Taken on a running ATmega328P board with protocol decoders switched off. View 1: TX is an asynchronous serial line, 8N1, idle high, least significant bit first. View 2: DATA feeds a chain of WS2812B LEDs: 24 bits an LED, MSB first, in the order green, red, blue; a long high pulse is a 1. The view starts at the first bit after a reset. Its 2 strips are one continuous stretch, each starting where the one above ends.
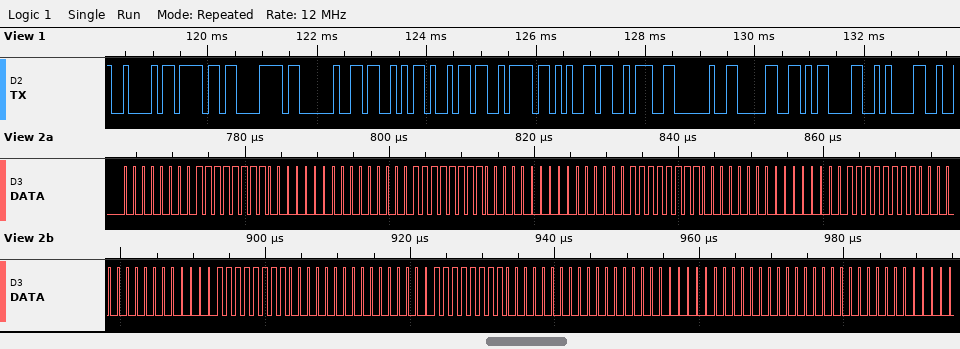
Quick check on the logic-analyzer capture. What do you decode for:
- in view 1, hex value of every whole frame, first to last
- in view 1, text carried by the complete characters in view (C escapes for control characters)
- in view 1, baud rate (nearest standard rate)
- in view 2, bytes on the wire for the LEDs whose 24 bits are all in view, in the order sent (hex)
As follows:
42 6F 78 20 53 69 7A 65 3A 20 30 0D 0A
"Box Size: 0\r\n"
9600 baud
00 FF 00 00 FF 00 00 FF 00 00 FF 00 00 FF 00 00 FF 00 00 00 00
